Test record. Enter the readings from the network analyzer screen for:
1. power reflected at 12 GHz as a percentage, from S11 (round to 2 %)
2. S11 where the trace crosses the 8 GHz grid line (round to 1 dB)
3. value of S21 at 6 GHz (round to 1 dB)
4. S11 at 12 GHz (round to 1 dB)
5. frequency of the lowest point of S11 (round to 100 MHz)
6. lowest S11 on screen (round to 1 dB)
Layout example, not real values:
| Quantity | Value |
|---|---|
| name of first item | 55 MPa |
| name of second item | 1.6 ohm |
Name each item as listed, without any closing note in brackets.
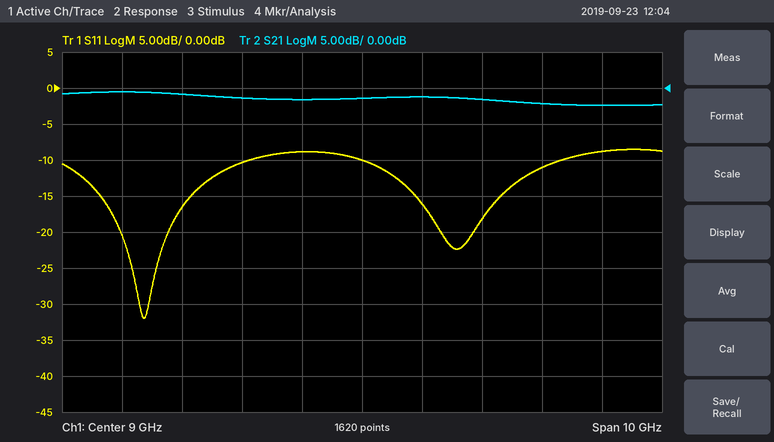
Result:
| Quantity | Value |
|---|---|
| power reflected at 12 GHz as a percentage, from S11 | 8 % |
| S11 where the trace crosses the 8 GHz grid line | -9 dB |
| value of S21 at 6 GHz | -1 dB |
| S11 at 12 GHz | -11 dB |
| frequency of the lowest point of S11 | 5.4 GHz |
| lowest S11 on screen | -32 dB |
